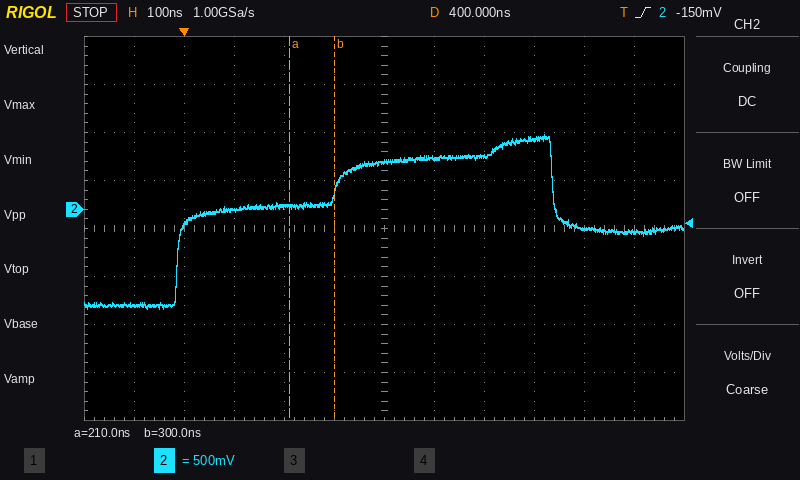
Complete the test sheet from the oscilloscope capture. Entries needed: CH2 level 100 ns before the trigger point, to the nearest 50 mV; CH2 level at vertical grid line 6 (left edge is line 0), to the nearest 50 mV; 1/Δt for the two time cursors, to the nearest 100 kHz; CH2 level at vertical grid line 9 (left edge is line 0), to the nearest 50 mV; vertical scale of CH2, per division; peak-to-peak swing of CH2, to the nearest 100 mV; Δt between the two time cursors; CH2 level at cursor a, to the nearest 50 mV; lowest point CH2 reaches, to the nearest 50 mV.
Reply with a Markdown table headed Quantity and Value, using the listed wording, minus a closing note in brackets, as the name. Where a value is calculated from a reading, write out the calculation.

| Quantity | Value |
|---|---|
| CH2 level 100 ns before the trigger point, to the nearest 50 mV | -1.00 V |
| CH2 level at vertical grid line 6 (left edge is line 0), to the nearest 50 mV | 500 mV |
| 1/Δt for the two time cursors, to the nearest 100 kHz | 1 / 90 ns ≈ 11.1 MHz |
| CH2 level at vertical grid line 9 (left edge is line 0), to the nearest 50 mV | 750 mV |
| vertical scale of CH2, per division | 500 mV |
| peak-to-peak swing of CH2, to the nearest 100 mV | 1.80 V |
| Δt between the two time cursors | 300 ns − (210 ns) = 90 ns |
| CH2 level at cursor a, to the nearest 50 mV | 50 mV |
| lowest point CH2 reaches, to the nearest 50 mV | -1.05 V |
